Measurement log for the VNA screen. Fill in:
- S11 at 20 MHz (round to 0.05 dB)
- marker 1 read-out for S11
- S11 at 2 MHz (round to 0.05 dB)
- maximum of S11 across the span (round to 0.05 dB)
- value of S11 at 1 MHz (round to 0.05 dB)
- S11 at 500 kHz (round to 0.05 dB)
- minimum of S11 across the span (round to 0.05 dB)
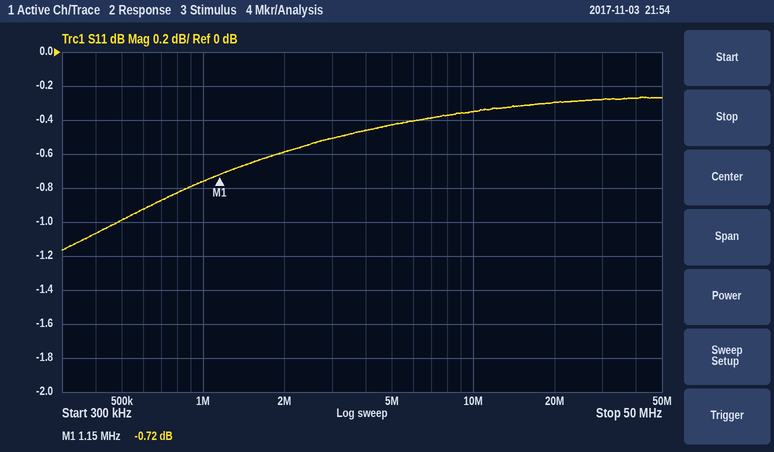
-0.30 dB
-0.72 dB
-0.60 dB
-0.25 dB
-0.75 dB
-1.00 dB
-1.15 dB
